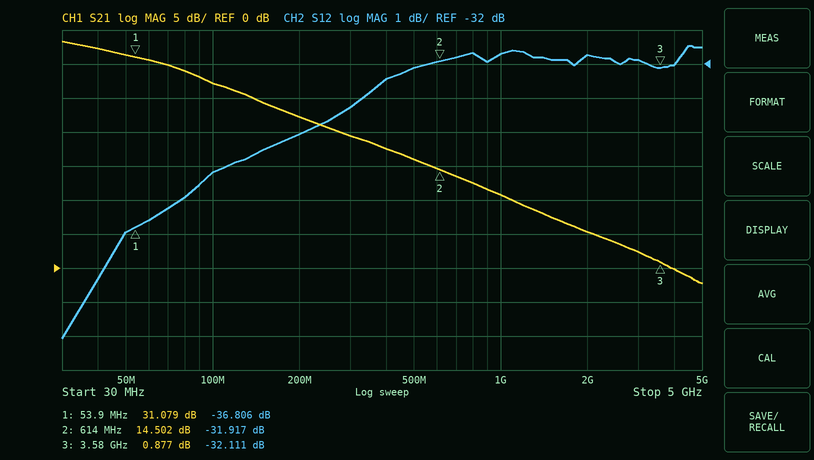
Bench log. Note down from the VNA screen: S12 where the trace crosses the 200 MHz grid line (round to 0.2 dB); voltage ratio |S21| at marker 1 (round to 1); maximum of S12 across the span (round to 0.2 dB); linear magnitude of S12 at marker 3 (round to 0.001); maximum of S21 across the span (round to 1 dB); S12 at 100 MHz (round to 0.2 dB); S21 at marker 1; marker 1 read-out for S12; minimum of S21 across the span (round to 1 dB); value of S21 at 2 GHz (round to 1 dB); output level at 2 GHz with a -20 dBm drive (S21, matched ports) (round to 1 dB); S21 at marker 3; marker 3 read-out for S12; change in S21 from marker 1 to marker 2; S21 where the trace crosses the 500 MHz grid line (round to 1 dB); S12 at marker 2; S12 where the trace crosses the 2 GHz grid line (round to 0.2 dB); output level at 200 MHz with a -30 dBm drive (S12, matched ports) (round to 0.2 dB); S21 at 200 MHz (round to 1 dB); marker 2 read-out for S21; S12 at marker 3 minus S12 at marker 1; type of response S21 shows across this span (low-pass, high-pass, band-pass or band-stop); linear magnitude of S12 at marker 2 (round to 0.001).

-34.0 dB
36
-31.4 dB
0.025
33 dB
-35.2 dB
31.079 dB
-36.806 dB
-2 dB
5 dB
-15 dBm
0.877 dB
-32.111 dB
-16.577 dB
16 dB
-31.917 dB
-31.8 dB
-64.0 dBm
22 dB
14.502 dB
4.695 dB
low-pass
0.025
